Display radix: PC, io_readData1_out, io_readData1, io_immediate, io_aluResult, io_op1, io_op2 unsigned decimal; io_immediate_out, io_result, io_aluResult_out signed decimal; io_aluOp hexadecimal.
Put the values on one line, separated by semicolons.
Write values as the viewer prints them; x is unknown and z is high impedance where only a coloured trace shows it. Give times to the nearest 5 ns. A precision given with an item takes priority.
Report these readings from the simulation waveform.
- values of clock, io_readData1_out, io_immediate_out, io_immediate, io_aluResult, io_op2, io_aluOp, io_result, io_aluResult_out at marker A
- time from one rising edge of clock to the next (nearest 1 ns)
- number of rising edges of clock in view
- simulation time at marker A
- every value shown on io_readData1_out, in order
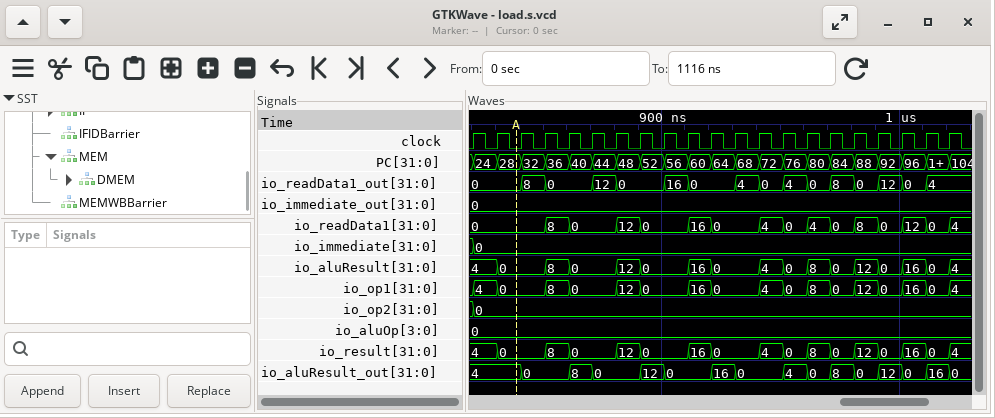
clock=0, io_readData1_out=0, io_immediate_out=0, io_immediate=0, io_aluResult=0, io_op2=0, io_aluOp=0, io_result=0, io_aluResult_out=4; 10 ns; 21; 840 ns; 0, 8, 0, 12, 0, 16, 0, 4, 0, 4, 0, 8, 0, 12, 0, 4
